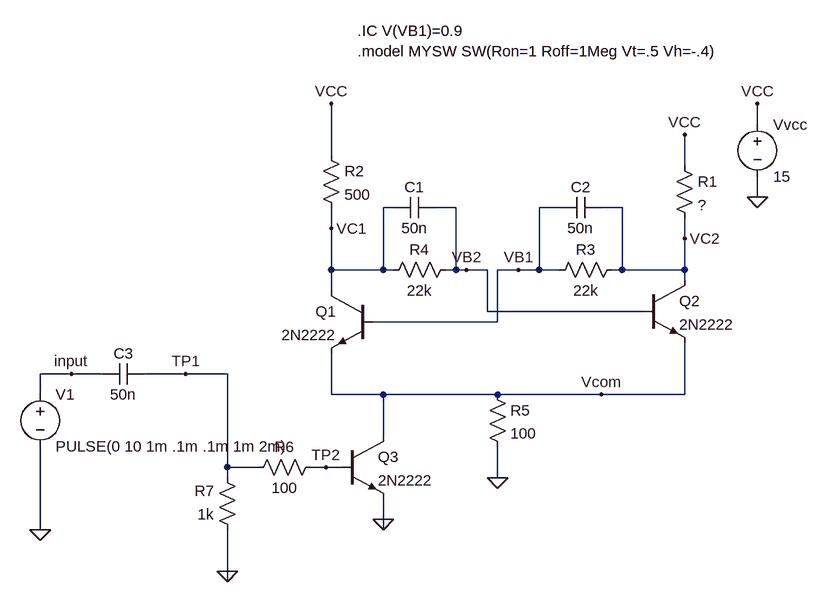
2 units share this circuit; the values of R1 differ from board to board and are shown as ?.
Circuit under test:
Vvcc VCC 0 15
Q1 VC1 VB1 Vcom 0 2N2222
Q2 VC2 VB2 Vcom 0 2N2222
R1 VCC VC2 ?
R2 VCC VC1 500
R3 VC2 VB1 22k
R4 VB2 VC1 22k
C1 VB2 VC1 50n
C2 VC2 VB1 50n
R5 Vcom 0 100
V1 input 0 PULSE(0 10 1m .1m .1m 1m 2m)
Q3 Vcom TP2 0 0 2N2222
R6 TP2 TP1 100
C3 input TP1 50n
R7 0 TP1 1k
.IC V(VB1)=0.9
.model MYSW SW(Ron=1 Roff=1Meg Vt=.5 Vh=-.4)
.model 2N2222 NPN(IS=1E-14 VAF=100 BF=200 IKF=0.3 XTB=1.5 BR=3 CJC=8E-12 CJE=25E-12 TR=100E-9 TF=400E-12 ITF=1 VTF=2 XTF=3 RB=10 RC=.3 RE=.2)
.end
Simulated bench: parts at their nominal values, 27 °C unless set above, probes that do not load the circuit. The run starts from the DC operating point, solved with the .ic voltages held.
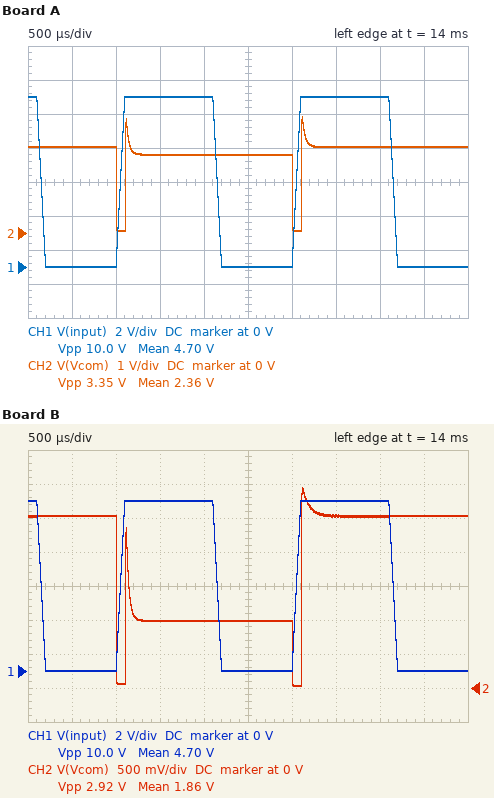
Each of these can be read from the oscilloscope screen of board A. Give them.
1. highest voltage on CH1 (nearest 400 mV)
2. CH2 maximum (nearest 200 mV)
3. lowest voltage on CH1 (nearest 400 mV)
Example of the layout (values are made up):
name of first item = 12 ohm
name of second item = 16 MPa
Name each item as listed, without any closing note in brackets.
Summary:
highest voltage on CH1 = 10.0 V
CH2 maximum = 3.4 V
lowest voltage on CH1 = 0 V
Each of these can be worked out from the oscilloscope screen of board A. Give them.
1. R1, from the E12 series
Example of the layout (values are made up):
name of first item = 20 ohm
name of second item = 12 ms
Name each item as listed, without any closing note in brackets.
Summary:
R1, from the E12 series = 560 Ω
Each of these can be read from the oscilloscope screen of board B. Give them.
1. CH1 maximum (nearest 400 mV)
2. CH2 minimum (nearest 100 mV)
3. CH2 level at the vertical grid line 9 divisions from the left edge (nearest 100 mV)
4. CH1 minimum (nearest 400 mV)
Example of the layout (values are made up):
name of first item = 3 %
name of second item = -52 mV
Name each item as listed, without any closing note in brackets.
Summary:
CH1 maximum = 10.0 V
CH2 minimum = 0 V
CH2 level at the vertical grid line 9 divisions from the left edge = 2.5 V
CH1 minimum = 0 V
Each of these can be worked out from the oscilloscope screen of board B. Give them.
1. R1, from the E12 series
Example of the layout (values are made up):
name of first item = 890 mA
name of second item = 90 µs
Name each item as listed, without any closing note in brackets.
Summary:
R1, from the E12 series = 1.5 kΩ
